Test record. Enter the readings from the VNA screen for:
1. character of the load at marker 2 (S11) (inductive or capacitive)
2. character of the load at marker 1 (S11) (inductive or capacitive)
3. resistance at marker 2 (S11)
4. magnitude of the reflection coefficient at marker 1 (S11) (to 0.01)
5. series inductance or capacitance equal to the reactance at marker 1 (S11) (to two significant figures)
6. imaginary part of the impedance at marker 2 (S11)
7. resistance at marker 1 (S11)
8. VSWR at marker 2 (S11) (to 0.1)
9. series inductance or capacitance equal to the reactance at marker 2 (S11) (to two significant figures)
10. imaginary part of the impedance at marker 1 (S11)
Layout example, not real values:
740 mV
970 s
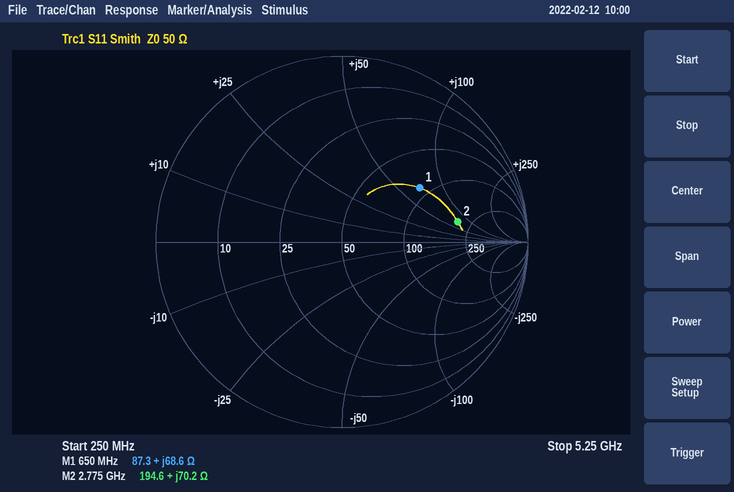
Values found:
inductive
inductive
194.6 Ω
0.51
17 nH
+70.2 Ω
87.3 Ω
4.4
4.0 nH
+68.6 Ω
